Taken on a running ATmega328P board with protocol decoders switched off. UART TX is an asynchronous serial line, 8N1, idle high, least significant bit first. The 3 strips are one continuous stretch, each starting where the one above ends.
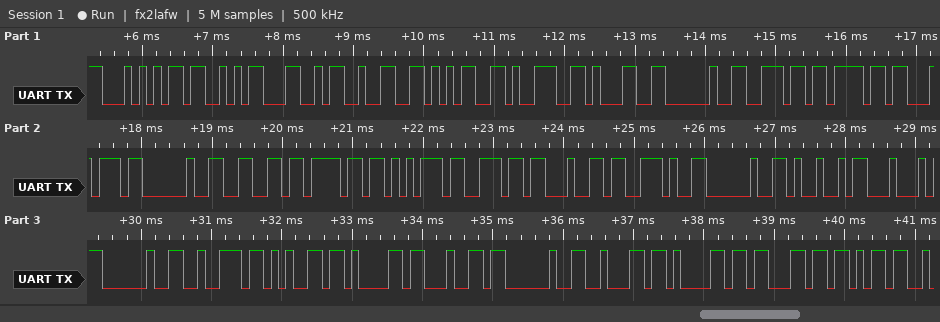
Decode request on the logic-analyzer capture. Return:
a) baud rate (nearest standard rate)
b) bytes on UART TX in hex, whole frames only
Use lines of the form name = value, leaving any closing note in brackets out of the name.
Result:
baud rate = 9600 baud
bytes on UART TX in hex, whole frames only = 54 53 4C 32 35 39 31 20 6E 6F 74 20 66 6F 75 6E 64 2E 20 49 44 20 72 65 61 64 20 62 61 63 6B
